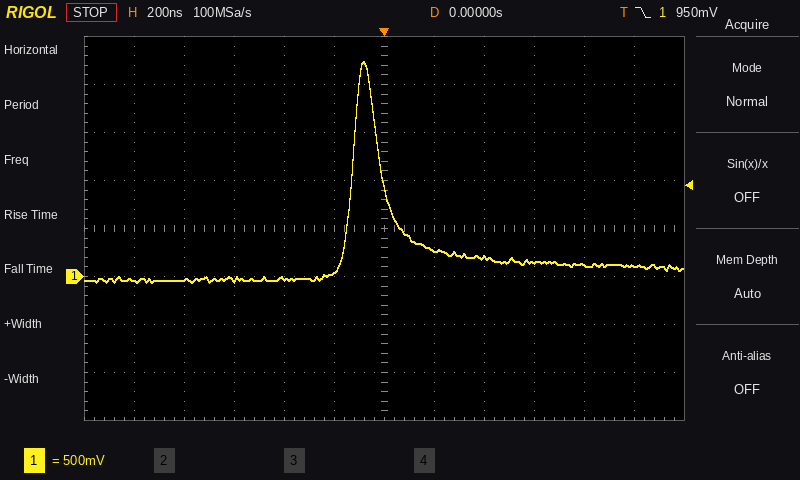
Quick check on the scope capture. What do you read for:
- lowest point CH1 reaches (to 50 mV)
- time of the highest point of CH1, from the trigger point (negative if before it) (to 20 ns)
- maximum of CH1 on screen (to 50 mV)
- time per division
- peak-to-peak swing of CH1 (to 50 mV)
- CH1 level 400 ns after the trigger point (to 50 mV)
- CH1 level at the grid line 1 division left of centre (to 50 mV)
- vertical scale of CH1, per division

-50 mV
-80 ns
2.25 V
200 ns
2.30 V
200 mV
50 mV
500 mV
